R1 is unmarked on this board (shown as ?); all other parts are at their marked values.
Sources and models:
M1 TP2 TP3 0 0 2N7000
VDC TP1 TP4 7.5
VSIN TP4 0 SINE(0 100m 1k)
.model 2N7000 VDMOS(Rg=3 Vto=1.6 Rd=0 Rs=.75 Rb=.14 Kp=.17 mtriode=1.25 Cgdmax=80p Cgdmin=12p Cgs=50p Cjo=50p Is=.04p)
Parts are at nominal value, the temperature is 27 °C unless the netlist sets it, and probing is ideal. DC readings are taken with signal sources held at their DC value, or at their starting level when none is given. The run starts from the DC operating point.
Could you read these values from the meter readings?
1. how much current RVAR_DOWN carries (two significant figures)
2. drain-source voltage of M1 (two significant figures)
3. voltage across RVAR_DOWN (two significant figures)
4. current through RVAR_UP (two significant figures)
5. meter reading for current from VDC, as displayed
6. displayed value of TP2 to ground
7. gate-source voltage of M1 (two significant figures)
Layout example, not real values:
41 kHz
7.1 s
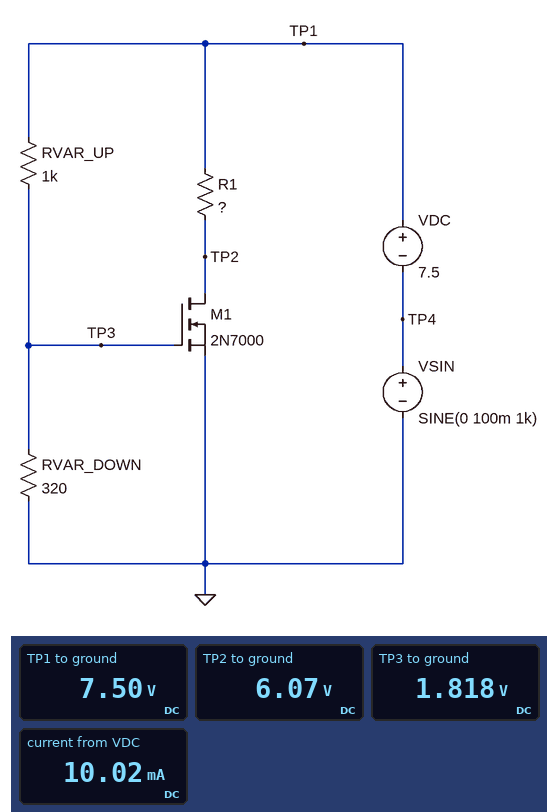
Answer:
5.7 mA
6.1 V
1.8 V
5.7 mA
10.02 mA
6.07 V
1.8 V
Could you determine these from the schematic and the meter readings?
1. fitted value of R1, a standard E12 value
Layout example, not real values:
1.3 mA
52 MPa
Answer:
330 Ω
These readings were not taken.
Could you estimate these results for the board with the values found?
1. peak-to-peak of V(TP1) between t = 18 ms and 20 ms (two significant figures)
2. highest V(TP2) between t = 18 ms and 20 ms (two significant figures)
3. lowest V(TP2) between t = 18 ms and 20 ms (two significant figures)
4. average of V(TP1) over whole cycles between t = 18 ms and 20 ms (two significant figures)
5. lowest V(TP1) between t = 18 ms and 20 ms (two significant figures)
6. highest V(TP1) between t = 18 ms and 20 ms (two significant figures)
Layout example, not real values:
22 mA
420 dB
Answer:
200 mV
6.2 V
5.9 V
7.5 V
7.4 V
7.6 V
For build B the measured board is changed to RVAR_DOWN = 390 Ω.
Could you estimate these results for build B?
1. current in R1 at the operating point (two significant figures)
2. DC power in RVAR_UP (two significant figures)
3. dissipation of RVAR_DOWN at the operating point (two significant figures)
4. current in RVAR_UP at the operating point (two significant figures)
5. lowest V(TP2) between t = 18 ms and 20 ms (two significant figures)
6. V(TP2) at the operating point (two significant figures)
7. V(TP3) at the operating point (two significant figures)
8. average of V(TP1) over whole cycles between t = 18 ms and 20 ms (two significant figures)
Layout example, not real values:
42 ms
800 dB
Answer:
20 mA
29 mW
11 mW
5.4 mA
360 mV
770 mV
2.1 V
7.5 V
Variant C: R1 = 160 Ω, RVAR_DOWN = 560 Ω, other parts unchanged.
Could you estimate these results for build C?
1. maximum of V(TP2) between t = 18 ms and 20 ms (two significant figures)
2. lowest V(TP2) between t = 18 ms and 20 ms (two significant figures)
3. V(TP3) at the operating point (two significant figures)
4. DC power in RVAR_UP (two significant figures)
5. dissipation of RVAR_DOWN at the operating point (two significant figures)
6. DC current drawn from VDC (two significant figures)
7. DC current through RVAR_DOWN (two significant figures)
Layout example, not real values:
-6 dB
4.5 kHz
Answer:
270 mV
260 mV
2.7 V
23 mW
13 mW
50 mA
4.8 mA
